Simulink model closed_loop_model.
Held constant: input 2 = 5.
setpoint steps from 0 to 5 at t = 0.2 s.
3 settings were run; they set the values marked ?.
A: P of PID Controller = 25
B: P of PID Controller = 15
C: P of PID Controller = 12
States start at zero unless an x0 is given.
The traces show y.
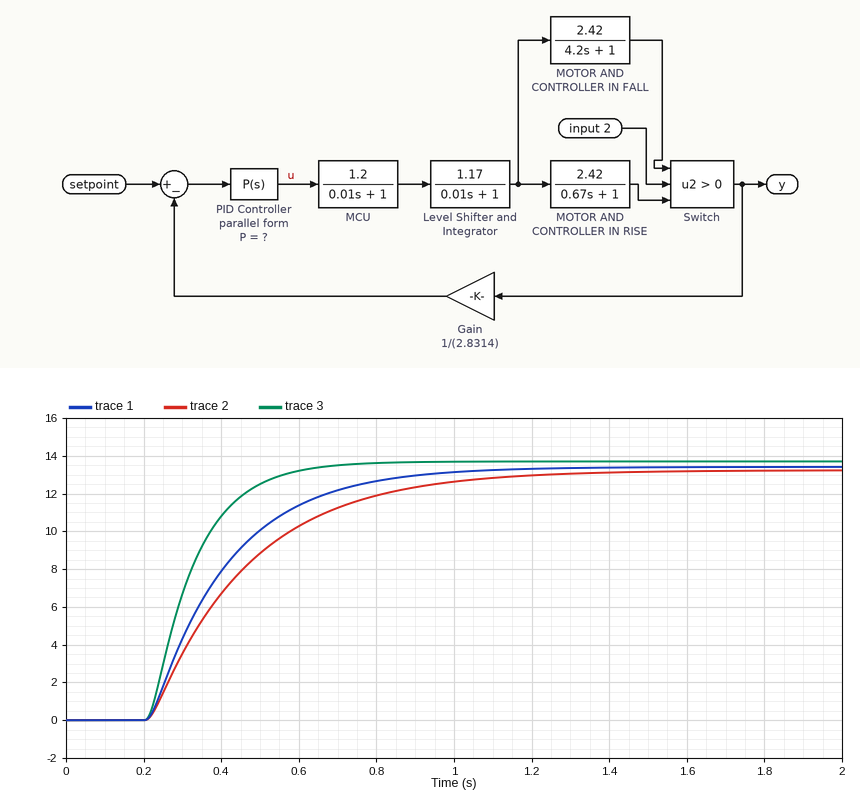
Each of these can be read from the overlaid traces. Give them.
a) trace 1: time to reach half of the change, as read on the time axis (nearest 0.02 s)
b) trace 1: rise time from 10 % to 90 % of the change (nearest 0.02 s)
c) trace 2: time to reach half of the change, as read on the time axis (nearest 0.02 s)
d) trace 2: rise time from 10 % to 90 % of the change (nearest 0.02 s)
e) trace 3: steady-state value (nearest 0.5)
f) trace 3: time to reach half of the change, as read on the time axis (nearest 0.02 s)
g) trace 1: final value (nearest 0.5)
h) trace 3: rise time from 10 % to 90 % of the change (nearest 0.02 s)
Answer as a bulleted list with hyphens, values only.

- 0.36 s
- 0.44 s
- 0.40 s
- 0.56 s
- 13.5
- 0.30 s
- 13.5
- 0.26 s
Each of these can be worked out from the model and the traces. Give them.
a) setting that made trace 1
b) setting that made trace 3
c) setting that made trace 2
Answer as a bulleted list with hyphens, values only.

- B
- A
- C
